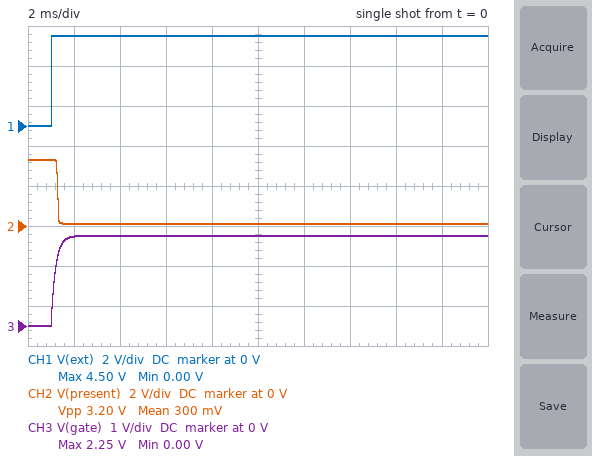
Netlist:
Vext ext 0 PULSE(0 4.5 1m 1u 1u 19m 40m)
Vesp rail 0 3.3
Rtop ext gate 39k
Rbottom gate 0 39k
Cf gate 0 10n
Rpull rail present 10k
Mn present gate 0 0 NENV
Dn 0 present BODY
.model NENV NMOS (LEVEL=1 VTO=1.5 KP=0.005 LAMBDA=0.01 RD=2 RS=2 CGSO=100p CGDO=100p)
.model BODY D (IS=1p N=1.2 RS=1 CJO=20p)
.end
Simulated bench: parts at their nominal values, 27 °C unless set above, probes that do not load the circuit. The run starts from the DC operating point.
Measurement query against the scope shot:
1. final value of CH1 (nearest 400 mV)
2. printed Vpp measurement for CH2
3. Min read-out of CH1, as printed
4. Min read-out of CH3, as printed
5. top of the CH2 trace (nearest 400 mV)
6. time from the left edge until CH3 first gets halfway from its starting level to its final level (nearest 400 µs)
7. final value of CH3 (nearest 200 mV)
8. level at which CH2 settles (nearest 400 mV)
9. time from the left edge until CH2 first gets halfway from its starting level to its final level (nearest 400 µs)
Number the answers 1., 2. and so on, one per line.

1. 4.4 V
2. 3.20 V
3. 0.00 V
4. 0.00 V
5. 3.2 V
6. 1.2 ms
7. 2.2 V
8. 0 V
9. 1.2 ms
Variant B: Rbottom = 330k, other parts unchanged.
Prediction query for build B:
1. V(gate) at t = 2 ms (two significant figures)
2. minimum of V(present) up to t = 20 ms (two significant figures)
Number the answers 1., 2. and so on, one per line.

1. 3.8 V
2. 27 mV
